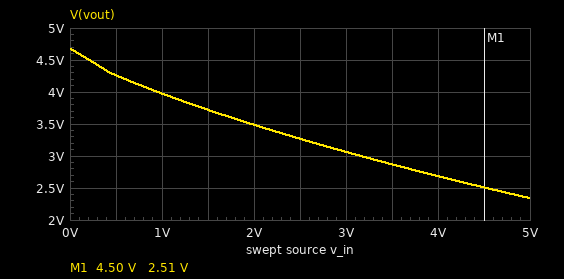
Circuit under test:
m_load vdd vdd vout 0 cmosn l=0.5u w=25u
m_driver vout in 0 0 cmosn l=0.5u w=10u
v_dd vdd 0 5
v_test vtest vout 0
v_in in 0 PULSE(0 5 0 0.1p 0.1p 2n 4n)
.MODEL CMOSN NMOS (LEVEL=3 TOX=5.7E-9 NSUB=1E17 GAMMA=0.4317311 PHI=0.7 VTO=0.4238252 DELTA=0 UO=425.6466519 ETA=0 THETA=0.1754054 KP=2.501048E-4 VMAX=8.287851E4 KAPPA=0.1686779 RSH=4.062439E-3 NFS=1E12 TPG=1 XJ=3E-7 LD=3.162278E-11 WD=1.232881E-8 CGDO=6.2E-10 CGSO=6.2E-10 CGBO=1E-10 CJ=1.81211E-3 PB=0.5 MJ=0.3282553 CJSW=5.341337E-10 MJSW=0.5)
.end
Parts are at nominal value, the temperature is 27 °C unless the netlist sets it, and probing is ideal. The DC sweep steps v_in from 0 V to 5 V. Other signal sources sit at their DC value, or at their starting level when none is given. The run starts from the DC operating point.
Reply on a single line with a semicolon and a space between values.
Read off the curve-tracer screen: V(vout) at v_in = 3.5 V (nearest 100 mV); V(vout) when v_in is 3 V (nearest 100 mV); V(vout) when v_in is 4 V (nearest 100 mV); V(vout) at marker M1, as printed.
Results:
2.9 V; 3.1 V; 2.7 V; 2.51 V
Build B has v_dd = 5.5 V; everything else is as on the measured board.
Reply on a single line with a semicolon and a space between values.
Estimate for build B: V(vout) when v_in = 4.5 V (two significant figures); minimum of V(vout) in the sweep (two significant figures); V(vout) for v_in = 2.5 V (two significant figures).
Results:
3.0 V; 2.8 V; 3.7 V
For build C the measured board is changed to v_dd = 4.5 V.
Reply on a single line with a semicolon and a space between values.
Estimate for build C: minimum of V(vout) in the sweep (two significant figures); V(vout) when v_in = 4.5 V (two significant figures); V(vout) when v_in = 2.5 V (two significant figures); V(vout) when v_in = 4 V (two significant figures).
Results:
1.9 V; 2.1 V; 2.8 V; 2.2 V
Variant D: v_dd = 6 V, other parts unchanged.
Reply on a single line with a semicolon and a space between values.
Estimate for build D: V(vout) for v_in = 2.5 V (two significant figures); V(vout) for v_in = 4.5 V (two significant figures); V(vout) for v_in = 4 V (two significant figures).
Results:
4.2 V; 3.4 V; 3.6 V
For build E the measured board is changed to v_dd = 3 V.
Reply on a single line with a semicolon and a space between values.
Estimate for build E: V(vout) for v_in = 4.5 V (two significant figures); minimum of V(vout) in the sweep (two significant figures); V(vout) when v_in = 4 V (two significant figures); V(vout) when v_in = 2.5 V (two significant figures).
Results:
910 mV; 850 mV; 990 mV; 1.4 V
